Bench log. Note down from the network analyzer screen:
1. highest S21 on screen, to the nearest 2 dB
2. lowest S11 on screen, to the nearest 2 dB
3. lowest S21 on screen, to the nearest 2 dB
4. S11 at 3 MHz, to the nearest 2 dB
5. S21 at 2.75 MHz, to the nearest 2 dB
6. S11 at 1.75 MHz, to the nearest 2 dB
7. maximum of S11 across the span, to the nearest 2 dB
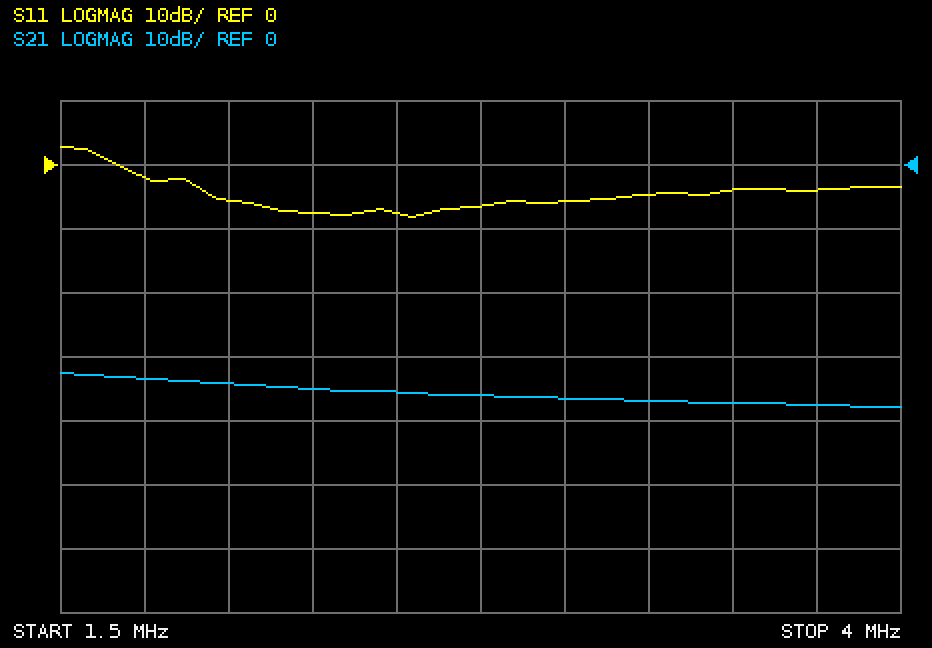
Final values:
-32 dB
-8 dB
-38 dB
-6 dB
-36 dB
-2 dB
2 dB
